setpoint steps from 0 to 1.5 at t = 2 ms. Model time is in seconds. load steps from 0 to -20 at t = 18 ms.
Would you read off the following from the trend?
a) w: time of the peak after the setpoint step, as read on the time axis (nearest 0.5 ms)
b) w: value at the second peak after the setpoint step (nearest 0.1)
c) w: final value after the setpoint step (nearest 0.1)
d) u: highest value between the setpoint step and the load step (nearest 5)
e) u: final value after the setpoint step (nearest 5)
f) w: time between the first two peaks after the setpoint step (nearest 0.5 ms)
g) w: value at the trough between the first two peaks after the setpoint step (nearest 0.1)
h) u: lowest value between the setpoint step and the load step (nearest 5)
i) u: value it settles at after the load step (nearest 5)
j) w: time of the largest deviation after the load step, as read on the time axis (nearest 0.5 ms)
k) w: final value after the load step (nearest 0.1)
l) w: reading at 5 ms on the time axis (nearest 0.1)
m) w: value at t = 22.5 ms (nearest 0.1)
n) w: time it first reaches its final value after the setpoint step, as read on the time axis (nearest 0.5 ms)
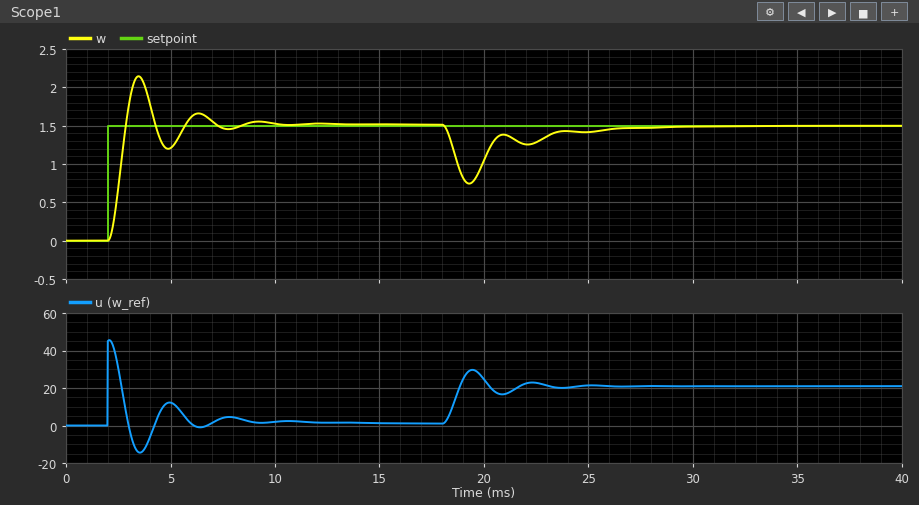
3.5 ms
1.7
1.5
45
0
3.0 ms
1.2
-15
20
19.5 ms
1.5
1.2
1.3
3.0 ms
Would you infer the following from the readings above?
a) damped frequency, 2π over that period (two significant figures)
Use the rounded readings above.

2.1 rad/ms
